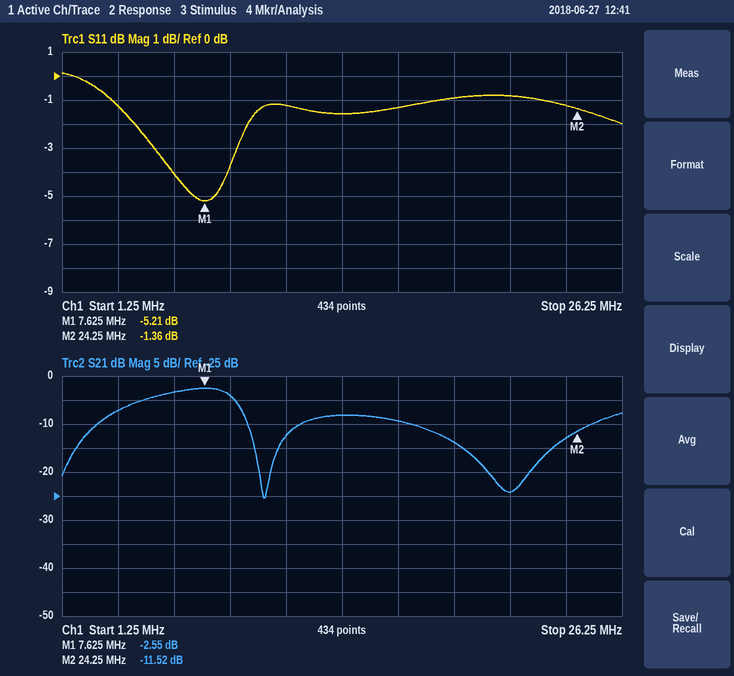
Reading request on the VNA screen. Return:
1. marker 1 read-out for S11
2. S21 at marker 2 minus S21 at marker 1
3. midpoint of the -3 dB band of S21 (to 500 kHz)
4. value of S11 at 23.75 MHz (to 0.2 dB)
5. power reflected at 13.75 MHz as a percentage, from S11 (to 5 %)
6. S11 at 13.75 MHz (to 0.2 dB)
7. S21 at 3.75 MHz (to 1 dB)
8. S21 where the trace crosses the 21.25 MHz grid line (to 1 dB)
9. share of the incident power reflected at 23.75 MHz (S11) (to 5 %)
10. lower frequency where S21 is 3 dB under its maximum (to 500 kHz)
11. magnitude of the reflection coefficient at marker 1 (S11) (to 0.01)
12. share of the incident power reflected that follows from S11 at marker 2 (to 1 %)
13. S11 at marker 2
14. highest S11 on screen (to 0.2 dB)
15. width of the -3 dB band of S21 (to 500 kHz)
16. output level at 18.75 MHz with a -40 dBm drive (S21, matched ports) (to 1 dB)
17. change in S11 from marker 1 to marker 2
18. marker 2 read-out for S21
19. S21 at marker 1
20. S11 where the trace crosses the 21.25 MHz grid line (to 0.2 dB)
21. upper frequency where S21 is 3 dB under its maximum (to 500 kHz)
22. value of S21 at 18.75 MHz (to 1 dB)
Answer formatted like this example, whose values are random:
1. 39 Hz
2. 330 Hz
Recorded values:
1. -5.21 dB
2. -8.97 dB
3. 7.0 MHz
4. -1.2 dB
5. 70 %
6. -1.6 dB
7. -7 dB
8. -24 dB
9. 75 %
10. 4.5 MHz
11. 0.55
12. 73 %
13. -1.36 dB
14. 0.2 dB
15. 4.5 MHz
16. -54 dBm
17. 3.85 dB
18. -11.52 dB
19. -2.55 dB
20. -0.8 dB
21. 9.0 MHz
22. -14 dB
